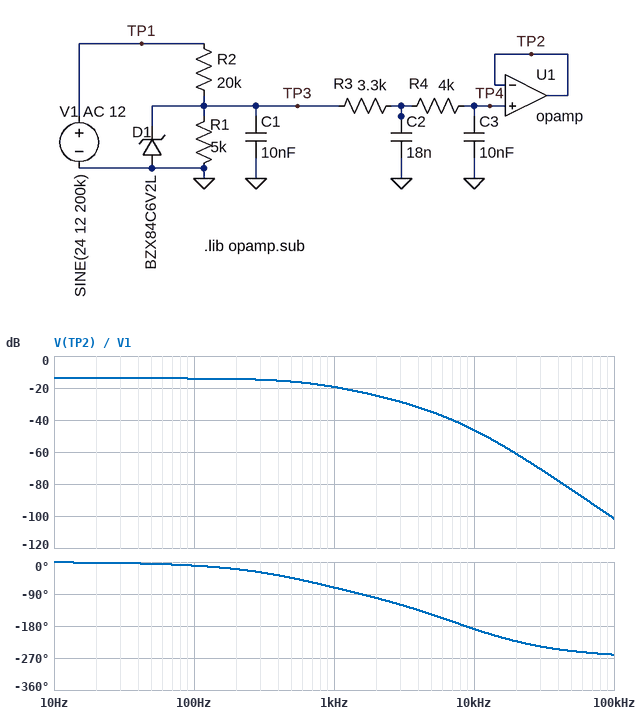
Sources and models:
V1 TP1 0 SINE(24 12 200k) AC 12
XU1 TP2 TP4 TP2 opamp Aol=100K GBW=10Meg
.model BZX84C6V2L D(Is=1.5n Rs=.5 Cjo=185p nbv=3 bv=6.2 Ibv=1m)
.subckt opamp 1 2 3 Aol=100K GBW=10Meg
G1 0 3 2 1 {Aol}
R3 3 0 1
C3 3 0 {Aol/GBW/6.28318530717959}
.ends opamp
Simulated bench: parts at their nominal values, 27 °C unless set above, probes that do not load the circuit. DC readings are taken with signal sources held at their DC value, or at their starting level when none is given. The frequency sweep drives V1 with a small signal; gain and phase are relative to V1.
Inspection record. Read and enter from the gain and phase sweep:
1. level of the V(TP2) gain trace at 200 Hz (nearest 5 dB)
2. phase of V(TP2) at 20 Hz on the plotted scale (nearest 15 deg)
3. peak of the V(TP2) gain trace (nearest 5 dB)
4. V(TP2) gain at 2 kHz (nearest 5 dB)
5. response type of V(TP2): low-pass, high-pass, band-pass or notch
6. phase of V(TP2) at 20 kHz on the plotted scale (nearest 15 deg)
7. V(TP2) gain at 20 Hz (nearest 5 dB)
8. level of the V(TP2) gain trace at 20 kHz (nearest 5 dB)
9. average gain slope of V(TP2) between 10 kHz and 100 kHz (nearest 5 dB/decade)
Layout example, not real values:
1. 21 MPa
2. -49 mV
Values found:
1. -15 dB
2. 0 deg
3. -15 dB
4. -25 dB
5. low-pass
6. -225 deg
7. -15 dB
8. -60 dB
9. -55 dB/decade
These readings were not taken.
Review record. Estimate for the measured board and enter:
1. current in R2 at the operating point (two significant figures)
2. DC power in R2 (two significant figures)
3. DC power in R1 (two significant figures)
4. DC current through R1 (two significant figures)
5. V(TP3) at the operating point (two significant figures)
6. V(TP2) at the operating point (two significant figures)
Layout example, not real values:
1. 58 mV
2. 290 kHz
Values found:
1. 960 µA
2. 18 mW
3. 4.6 mW
4. 960 µA
5. 4.8 V
6. 4.8 V
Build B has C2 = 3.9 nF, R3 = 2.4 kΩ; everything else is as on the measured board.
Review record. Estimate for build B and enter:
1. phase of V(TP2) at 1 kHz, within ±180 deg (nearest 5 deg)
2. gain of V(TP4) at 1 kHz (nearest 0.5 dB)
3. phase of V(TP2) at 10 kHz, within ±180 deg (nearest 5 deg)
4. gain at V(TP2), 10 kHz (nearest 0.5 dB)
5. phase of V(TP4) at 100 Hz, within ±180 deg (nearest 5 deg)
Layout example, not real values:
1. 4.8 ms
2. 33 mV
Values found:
1. -50 deg
2. -16.5 dB
3. -155 deg
4. -38.0 dB
5. -5 deg
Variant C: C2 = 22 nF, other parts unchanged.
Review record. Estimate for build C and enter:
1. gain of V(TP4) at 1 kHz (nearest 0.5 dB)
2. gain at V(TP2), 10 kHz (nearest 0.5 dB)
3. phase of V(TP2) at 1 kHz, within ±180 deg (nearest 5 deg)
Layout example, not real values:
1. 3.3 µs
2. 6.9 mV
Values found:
1. -20.0 dB
2. -47.5 dB
3. -75 deg
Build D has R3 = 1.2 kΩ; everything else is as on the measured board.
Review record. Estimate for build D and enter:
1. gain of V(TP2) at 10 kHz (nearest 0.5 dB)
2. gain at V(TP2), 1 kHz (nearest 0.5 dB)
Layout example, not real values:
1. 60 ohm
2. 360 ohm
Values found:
1. -42.5 dB
2. -18.0 dB
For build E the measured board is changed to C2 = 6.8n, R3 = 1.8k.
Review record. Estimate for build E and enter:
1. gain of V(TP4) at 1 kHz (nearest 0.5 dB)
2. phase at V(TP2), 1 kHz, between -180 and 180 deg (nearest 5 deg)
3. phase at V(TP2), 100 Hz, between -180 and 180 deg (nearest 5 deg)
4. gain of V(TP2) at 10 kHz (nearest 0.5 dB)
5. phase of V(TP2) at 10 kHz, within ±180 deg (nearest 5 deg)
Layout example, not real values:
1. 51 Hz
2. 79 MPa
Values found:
1. -17.0 dB
2. -55 deg
3. -5 deg
4. -39.0 dB
5. -160 deg
